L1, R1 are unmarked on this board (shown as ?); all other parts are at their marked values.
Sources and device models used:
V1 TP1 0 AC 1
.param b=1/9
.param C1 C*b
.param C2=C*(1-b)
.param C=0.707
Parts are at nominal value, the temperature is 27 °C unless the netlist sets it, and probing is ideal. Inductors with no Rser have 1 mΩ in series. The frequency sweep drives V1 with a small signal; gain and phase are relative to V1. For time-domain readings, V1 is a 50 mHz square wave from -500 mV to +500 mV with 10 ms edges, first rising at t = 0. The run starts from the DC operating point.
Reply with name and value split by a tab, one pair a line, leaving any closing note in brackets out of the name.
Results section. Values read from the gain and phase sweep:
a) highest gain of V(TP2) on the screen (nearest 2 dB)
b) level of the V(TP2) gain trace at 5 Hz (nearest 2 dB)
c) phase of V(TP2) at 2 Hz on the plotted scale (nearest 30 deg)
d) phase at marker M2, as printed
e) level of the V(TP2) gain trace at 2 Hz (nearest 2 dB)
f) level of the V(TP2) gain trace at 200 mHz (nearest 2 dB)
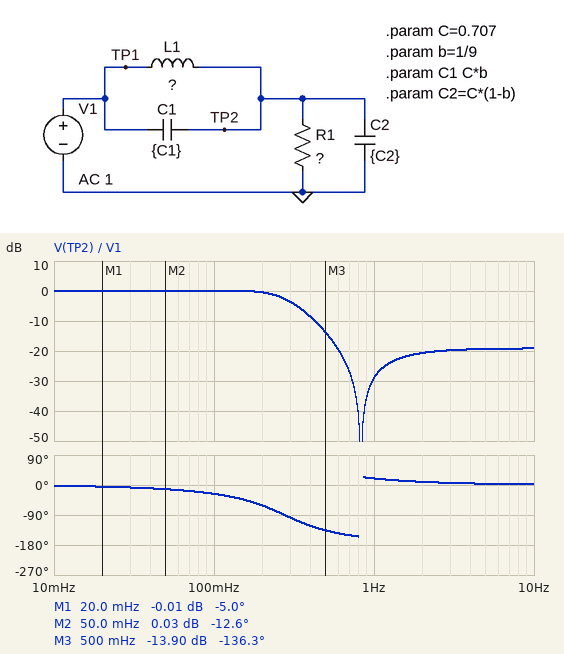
highest gain of V(TP2) on the screen	0 dB
level of the V(TP2) gain trace at 5 Hz	-20 dB
phase of V(TP2) at 2 Hz on the plotted scale	0 deg
phase at marker M2, as printed	-12.6 deg
level of the V(TP2) gain trace at 2 Hz	-20 dB
level of the V(TP2) gain trace at 200 mHz	0 dB
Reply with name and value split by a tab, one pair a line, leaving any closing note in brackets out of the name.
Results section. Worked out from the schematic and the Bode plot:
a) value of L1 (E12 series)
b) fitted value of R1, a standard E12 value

value of L1	470 mH
fitted value of R1, a standard E12 value	0.68 Ω
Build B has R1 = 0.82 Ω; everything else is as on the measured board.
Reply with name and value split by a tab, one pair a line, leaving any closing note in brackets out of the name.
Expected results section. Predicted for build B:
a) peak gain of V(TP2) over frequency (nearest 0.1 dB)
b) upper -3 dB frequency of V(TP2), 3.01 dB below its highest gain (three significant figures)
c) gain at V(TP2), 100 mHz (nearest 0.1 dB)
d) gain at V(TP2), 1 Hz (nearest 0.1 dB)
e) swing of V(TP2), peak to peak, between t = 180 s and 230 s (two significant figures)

peak gain of V(TP2) over frequency	0.8 dB
upper -3 dB frequency of V(TP2), 3.01 dB below its highest gain	304 mHz
gain at V(TP2), 100 mHz	0.4 dB
gain at V(TP2), 1 Hz	-28.8 dB
swing of V(TP2), peak to peak, between t = 180 s and 230 s	1.3 V
